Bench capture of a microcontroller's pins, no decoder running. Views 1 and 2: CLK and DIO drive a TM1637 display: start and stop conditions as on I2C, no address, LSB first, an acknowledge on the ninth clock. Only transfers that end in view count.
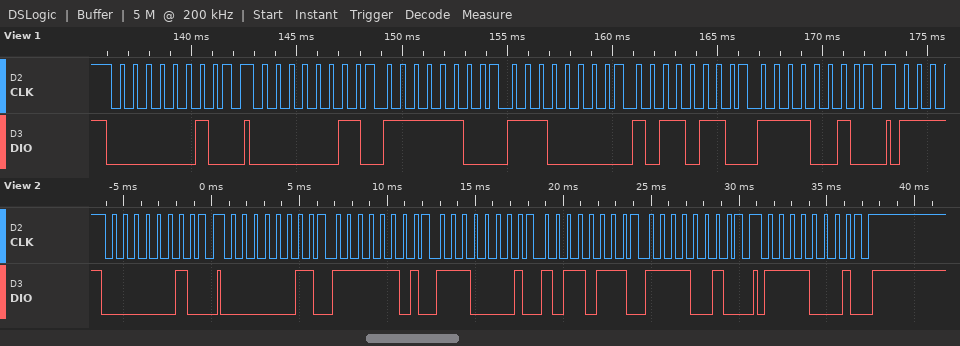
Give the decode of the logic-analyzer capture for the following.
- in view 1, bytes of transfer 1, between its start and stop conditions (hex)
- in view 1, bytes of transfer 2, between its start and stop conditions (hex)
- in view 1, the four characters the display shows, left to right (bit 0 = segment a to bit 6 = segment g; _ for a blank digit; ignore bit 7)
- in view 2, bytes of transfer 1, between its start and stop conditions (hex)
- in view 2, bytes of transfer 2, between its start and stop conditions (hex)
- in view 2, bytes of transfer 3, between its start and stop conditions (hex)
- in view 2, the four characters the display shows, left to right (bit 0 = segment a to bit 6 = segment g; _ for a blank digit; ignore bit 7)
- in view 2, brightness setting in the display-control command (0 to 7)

40
C0 3F 07 6D 4F
0753
40
C0 BF 87 ED 4F
8F
0753
7
